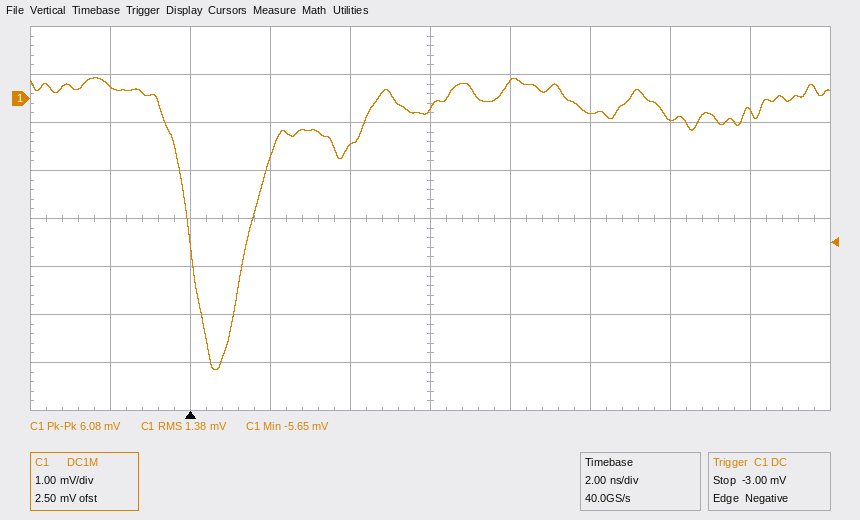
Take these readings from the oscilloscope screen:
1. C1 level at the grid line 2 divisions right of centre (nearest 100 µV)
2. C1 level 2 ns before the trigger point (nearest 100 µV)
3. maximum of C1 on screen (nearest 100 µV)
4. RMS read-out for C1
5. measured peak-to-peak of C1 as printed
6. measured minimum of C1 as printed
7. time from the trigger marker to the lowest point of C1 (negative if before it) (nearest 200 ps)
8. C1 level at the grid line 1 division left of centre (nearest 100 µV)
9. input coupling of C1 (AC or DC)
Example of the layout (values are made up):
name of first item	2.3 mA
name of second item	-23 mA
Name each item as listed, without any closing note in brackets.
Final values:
C1 level at the grid line 2 divisions right of centre	-300 µV
C1 level 2 ns before the trigger point	300 µV
maximum of C1 on screen	400 µV
RMS read-out for C1	1.38 mV
measured peak-to-peak of C1 as printed	6.08 mV
measured minimum of C1 as printed	-5.65 mV
time from the trigger marker to the lowest point of C1 (negative if before it)	+600 ps
C1 level at the grid line 1 division left of centre	-1.0 mV
input coupling of C1	DC
